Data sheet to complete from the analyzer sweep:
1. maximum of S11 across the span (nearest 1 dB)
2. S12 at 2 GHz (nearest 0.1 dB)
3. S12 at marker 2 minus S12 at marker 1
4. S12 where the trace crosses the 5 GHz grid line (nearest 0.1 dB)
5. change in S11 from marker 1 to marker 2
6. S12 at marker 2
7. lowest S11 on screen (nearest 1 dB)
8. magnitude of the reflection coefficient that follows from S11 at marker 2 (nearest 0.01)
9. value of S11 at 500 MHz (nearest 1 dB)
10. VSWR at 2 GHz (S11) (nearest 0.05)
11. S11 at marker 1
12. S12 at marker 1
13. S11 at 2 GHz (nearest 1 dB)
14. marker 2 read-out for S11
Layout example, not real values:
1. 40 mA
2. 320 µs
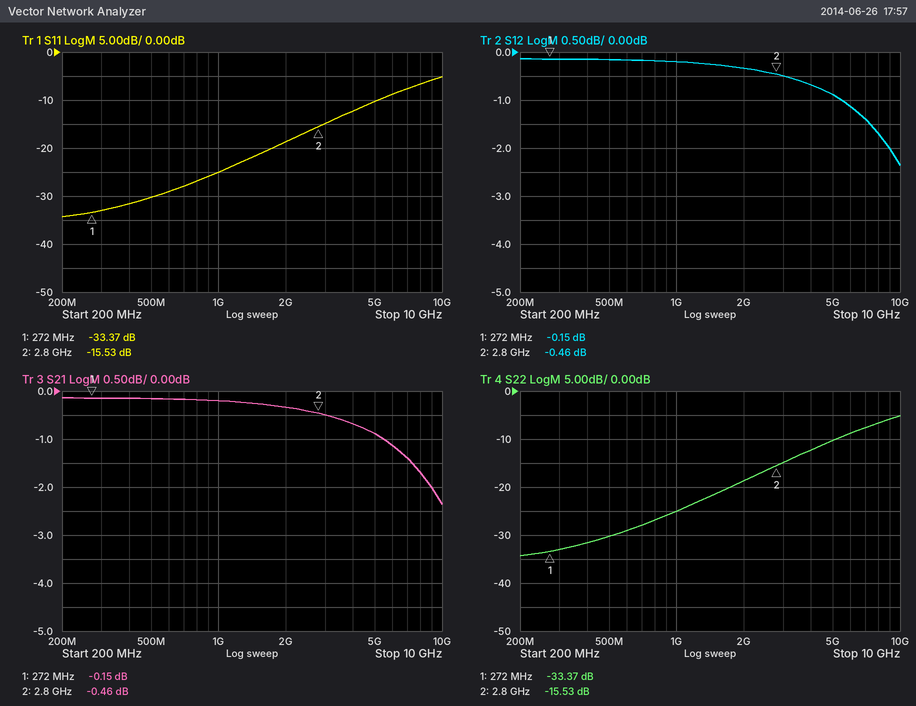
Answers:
1. -5 dB
2. -0.3 dB
3. -0.31 dB
4. -0.9 dB
5. 17.84 dB
6. -0.46 dB
7. -34 dB
8. 0.17
9. -30 dB
10. 1.25
11. -33.37 dB
12. -0.15 dB
13. -19 dB
14. -15.53 dB
